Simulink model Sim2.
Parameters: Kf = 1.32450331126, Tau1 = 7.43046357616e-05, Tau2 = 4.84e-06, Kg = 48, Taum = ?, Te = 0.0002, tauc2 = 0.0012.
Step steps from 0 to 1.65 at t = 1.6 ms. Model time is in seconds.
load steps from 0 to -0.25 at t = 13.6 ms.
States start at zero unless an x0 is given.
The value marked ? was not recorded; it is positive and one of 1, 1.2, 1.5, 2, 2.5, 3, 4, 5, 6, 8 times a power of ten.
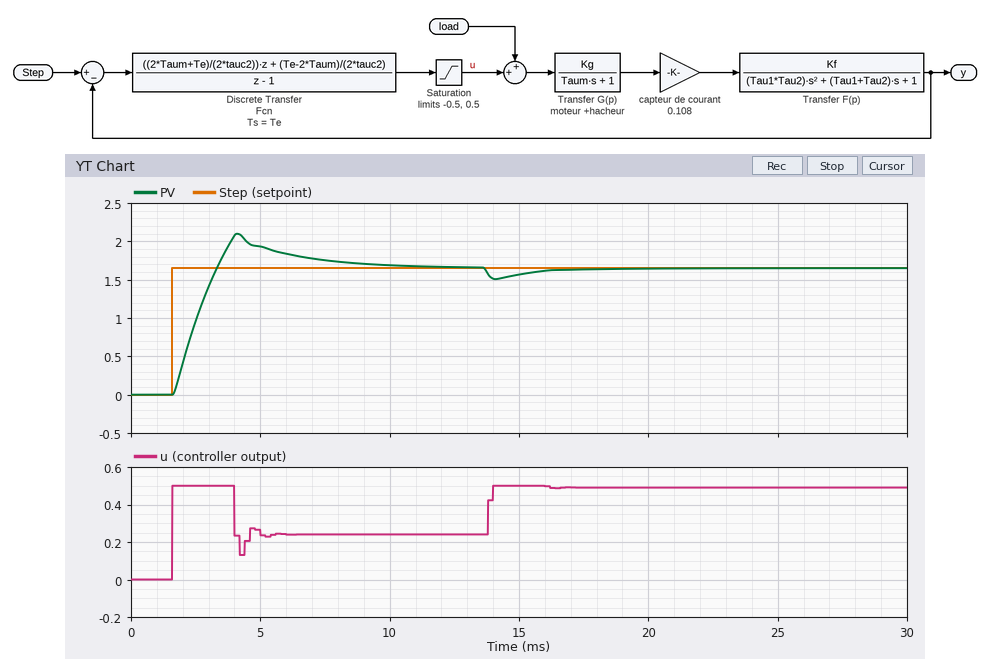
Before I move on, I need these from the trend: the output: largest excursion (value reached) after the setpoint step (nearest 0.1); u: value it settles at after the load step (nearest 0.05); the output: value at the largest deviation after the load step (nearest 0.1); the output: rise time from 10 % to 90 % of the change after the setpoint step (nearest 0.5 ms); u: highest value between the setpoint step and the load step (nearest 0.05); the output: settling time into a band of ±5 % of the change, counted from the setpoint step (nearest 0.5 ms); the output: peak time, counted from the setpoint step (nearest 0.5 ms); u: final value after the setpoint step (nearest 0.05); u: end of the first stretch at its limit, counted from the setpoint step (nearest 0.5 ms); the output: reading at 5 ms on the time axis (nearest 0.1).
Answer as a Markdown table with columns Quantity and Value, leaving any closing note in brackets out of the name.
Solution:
| Quantity | Value |
|---|---|
| the output: largest excursion (value reached) after the setpoint step | 2.1 |
| u: value it settles at after the load step | 0.50 |
| the output: value at the largest deviation after the load step | 1.5 |
| the output: rise time from 10 % to 90 % of the change after the setpoint step | 1.5 ms |
| u: highest value between the setpoint step and the load step | 0.50 |
| the output: settling time into a band of ±5 % of the change, counted from the setpoint step | 6.5 ms |
| the output: peak time, counted from the setpoint step | 2.5 ms |
| u: final value after the setpoint step | 0.25 |
| u: end of the first stretch at its limit, counted from the setpoint step | 2.5 ms |
| the output: reading at 5 ms on the time axis | 1.9 |
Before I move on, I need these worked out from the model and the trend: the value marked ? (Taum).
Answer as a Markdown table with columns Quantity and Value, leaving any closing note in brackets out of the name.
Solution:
| Quantity | Value |
|---|---|
| the value marked ? | 0.0025 |
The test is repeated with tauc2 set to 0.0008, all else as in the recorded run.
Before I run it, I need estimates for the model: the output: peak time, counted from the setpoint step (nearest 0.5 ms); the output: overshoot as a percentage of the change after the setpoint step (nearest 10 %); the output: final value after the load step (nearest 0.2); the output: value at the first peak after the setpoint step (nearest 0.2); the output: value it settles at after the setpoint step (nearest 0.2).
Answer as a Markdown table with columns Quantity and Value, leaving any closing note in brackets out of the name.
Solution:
| Quantity | Value |
|---|---|
| the output: peak time, counted from the setpoint step | 2.5 ms |
| the output: overshoot as a percentage of the change after the setpoint step | 30 % |
| the output: final value after the load step | 1.6 |
| the output: value at the first peak after the setpoint step | 2.2 |
| the output: value it settles at after the setpoint step | 1.6 |
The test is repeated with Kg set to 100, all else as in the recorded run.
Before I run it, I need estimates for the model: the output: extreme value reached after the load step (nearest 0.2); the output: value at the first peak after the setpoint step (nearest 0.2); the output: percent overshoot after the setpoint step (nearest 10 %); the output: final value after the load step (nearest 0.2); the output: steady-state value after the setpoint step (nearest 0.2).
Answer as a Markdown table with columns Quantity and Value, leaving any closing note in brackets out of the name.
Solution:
| Quantity | Value |
|---|---|
| the output: extreme value reached after the load step | 1.4 |
| the output: value at the first peak after the setpoint step | 2.2 |
| the output: percent overshoot after the setpoint step | 30 % |
| the output: final value after the load step | 1.6 |
| the output: steady-state value after the setpoint step | 1.6 |
